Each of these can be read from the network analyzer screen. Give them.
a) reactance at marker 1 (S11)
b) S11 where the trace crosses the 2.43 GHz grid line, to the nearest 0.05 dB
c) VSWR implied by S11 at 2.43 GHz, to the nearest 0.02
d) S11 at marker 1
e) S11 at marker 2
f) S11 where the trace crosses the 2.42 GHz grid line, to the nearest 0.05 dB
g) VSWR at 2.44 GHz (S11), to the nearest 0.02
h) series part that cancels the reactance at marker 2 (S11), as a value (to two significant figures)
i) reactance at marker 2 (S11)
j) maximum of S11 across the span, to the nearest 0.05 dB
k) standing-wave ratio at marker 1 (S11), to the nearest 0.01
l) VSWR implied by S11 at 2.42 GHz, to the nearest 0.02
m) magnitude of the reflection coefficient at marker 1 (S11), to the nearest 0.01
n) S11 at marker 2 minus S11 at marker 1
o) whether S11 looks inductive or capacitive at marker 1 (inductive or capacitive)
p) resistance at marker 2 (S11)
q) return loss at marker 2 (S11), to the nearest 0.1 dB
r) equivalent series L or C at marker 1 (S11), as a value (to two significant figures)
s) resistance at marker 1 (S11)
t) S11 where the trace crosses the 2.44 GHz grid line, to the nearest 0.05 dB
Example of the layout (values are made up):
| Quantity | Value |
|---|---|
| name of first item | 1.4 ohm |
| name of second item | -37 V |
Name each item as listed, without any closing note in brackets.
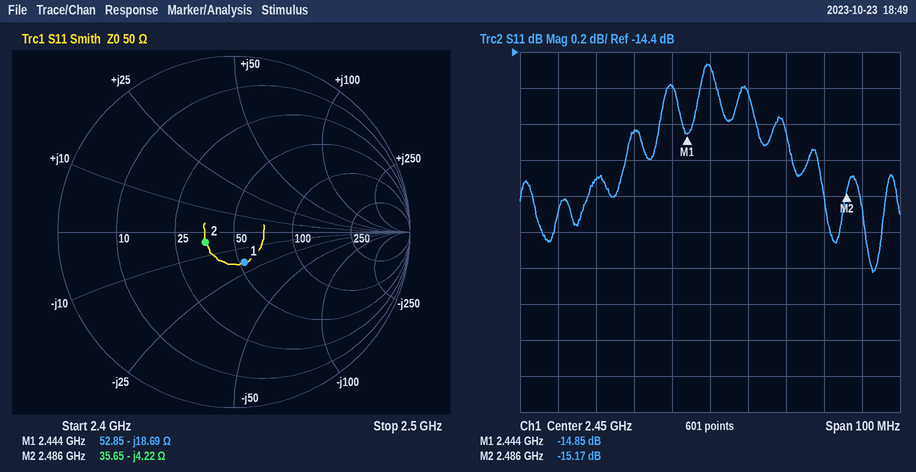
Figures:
| Quantity | Value |
|---|---|
| reactance at marker 1 | -18.69 Ω |
| S11 where the trace crosses the 2.43 GHz grid line, to the nearest 0.05 dB | -14.85 dB |
| VSWR implied by S11 at 2.43 GHz, to the nearest 0.02 | 1.44 |
| S11 at marker 1 | -14.85 dB |
| S11 at marker 2 | -15.17 dB |
| S11 where the trace crosses the 2.42 GHz grid line, to the nearest 0.05 dB | -15.10 dB |
| VSWR at 2.44 GHz (S11), to the nearest 0.02 | 1.46 |
| series part that cancels the reactance at marker 2 (S11), as a value | 270 pH |
| reactance at marker 2 | -4.22 Ω |
| maximum of S11 across the span, to the nearest 0.05 dB | -14.45 dB |
| standing-wave ratio at marker 1 (S11), to the nearest 0.01 | 1.44 |
| VSWR implied by S11 at 2.42 GHz, to the nearest 0.02 | 1.42 |
| magnitude of the reflection coefficient at marker 1 (S11), to the nearest 0.01 | 0.18 |
| S11 at marker 2 minus S11 at marker 1 | -0.32 dB |
| whether S11 looks inductive or capacitive at marker 1 | capacitive |
| resistance at marker 2 | 35.65 Ω |
| return loss at marker 2 (S11), to the nearest 0.1 dB | 15.2 dB |
| equivalent series L or C at marker 1 (S11), as a value | 3.5 pF |
| resistance at marker 1 | 52.85 Ω |
| S11 where the trace crosses the 2.44 GHz grid line, to the nearest 0.05 dB | -14.60 dB |
